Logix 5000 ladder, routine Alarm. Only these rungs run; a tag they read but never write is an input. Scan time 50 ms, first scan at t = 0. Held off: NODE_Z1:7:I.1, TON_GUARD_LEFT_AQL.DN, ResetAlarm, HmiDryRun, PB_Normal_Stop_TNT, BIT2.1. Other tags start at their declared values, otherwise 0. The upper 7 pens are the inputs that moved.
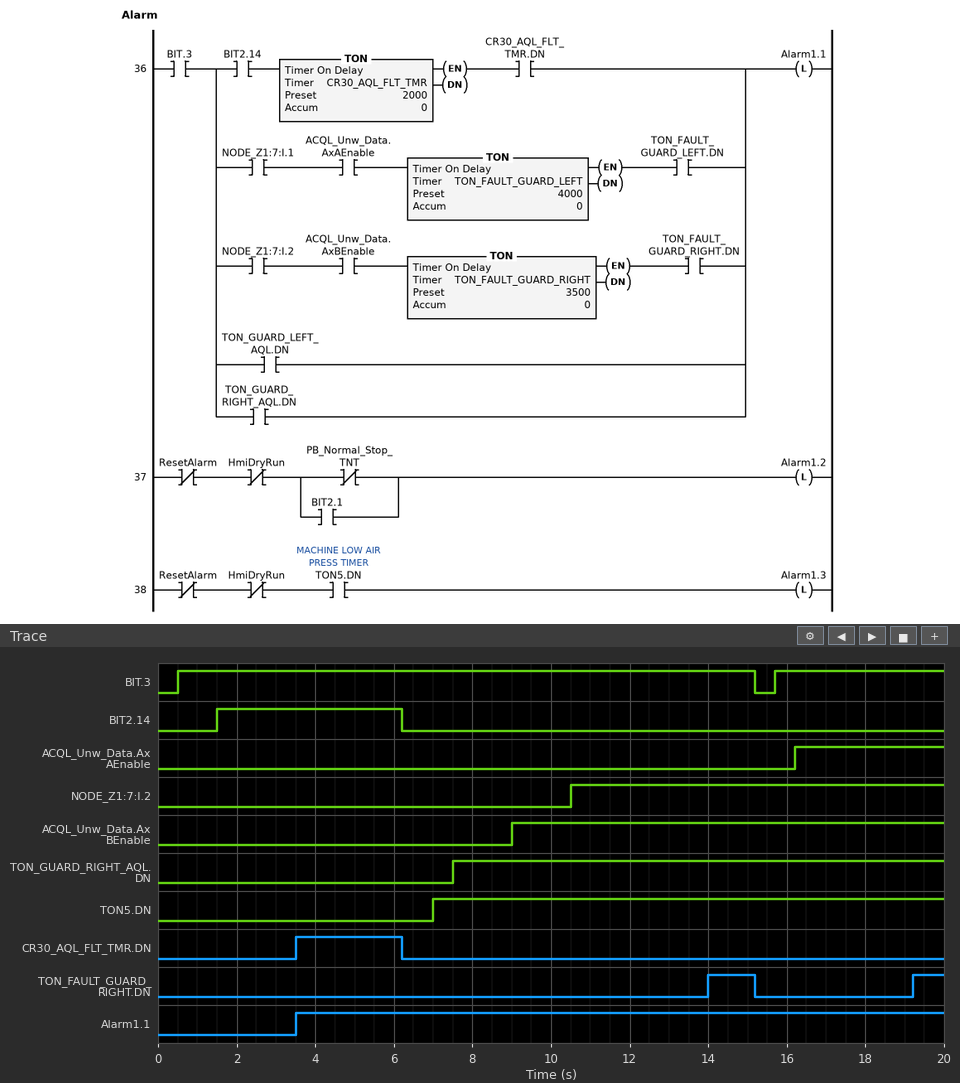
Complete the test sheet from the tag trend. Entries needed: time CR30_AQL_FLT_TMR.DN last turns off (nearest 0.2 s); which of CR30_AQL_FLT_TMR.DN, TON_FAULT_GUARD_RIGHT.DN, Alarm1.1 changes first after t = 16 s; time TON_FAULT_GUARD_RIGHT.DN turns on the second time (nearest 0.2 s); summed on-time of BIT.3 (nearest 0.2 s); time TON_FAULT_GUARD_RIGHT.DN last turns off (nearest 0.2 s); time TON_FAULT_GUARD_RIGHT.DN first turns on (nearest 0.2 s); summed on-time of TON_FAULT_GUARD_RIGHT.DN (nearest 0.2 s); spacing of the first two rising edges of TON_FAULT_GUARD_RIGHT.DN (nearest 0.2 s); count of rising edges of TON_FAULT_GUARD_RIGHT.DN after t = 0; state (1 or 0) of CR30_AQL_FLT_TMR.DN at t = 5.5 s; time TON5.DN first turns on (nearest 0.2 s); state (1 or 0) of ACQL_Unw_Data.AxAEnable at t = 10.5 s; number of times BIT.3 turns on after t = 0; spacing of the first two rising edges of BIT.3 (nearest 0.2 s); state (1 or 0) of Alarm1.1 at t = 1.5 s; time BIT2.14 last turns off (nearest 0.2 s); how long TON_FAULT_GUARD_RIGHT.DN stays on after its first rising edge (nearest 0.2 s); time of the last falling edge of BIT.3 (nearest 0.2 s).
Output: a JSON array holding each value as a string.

["6.2 s", "TON_FAULT_GUARD_RIGHT.DN", "19.2 s", "19.0 s", "15.2 s", "14.0 s", "2.0 s", "5.2 s", "2", "1", "7.0 s", "0", "2", "15.2 s", "0", "6.2 s", "1.2 s", "15.2 s"]
